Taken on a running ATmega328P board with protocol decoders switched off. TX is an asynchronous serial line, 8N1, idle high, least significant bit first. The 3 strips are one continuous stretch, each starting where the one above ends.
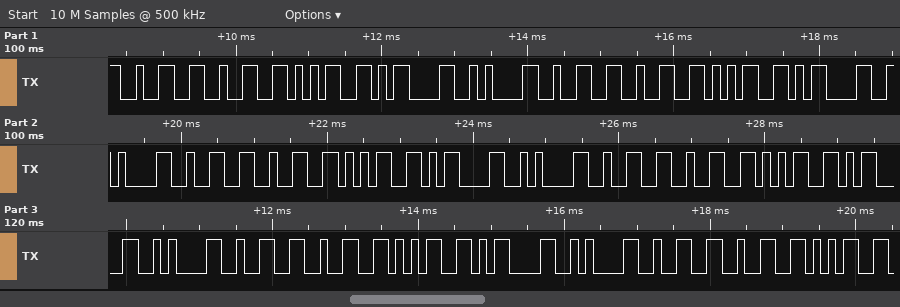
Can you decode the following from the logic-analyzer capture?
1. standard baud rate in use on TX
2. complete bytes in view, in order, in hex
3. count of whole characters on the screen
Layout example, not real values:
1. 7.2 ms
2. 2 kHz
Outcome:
1. 9600 baud
2. 0x32 0x32 0x35 0x0D 0x0A 0x32 0x32 0x35 0x0D 0x0A 0x32 0x32 0x35 0x0D 0x0A 0x32 0x32 0x35 0x0D 0x0A 0x32 0x32 0x35 0x0D 0x0A 0x32 0x32 0x35
3. 28
